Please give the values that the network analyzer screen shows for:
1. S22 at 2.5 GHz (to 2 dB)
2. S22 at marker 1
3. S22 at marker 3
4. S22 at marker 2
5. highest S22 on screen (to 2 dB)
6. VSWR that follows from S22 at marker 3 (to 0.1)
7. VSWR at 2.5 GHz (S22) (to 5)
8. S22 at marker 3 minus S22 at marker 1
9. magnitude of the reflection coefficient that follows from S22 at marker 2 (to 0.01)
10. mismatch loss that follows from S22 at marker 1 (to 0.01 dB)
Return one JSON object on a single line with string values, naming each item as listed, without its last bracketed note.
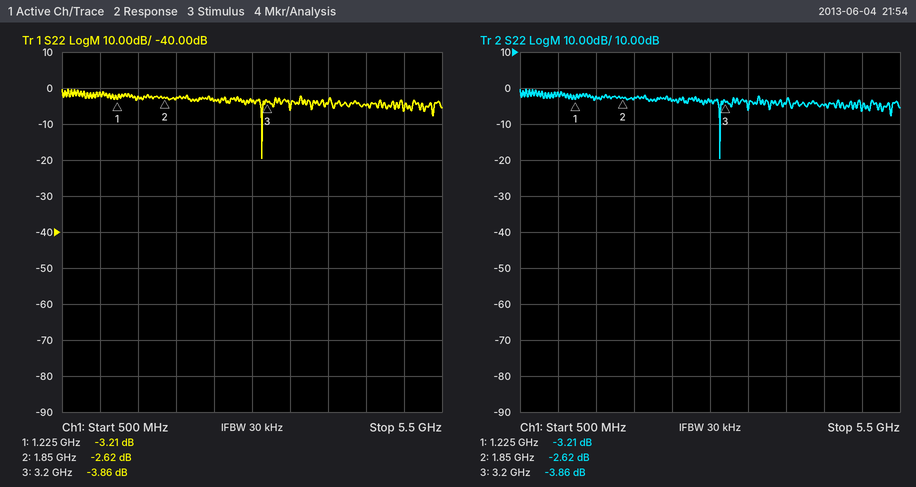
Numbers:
{"S22 at 2.5 GHz": "-4 dB", "S22 at marker 1": "-3.21 dB", "S22 at marker 3": "-3.86 dB", "S22 at marker 2": "-2.62 dB", "highest S22 on screen": "0 dB", "VSWR that follows from S22 at marker 3": "4.6", "VSWR at 2.5 GHz (S22)": "5", "S22 at marker 3 minus S22 at marker 1": "-0.65 dB", "magnitude of the reflection coefficient that follows from S22 at marker 2": "0.74", "mismatch loss that follows from S22 at marker 1": "2.82 dB"}
